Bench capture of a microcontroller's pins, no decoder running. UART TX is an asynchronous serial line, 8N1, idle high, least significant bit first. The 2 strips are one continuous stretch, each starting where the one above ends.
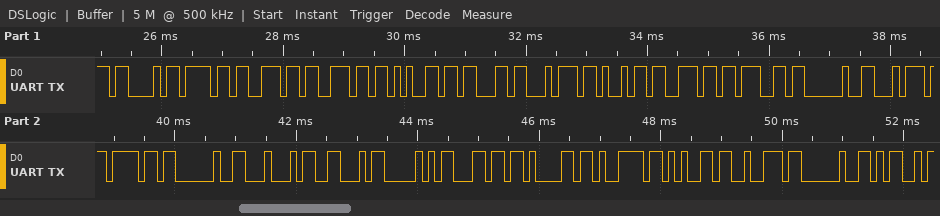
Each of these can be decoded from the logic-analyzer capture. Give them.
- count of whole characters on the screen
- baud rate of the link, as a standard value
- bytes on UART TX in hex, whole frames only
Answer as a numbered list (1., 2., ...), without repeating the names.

1. 24
2. 9600 baud
3. 43 6F 6E 6E 65 63 74 69 6E 67 20 74 6F 20 44 46 50 6C 61 79 65 72 20 4D
